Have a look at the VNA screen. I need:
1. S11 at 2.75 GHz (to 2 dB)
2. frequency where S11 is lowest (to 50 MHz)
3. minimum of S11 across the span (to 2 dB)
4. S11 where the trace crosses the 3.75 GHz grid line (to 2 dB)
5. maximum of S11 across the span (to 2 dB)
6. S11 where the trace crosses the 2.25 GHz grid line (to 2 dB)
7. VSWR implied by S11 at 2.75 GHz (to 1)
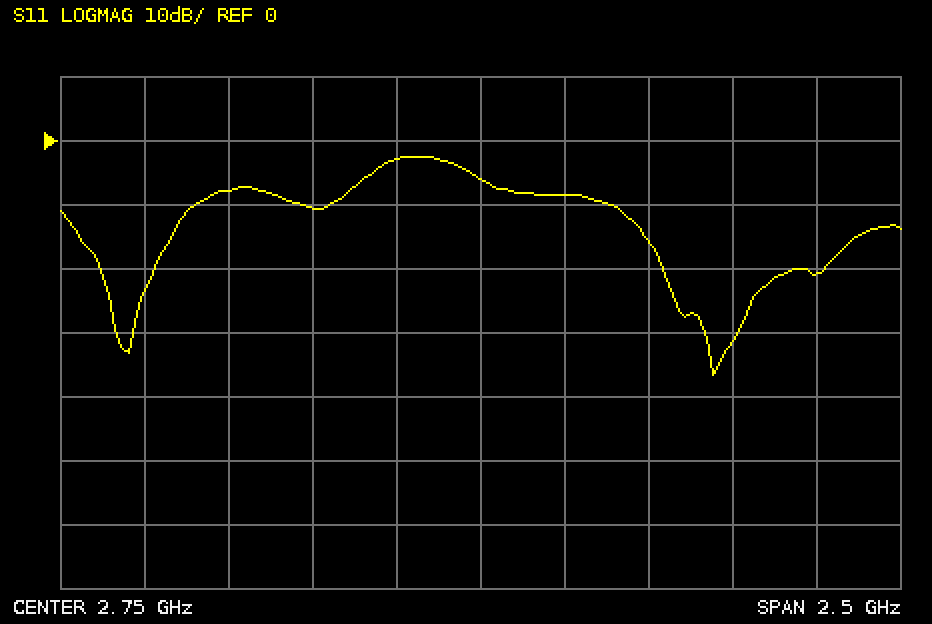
-6 dB
3.45 GHz
-36 dB
-20 dB
-2 dB
-10 dB
3
